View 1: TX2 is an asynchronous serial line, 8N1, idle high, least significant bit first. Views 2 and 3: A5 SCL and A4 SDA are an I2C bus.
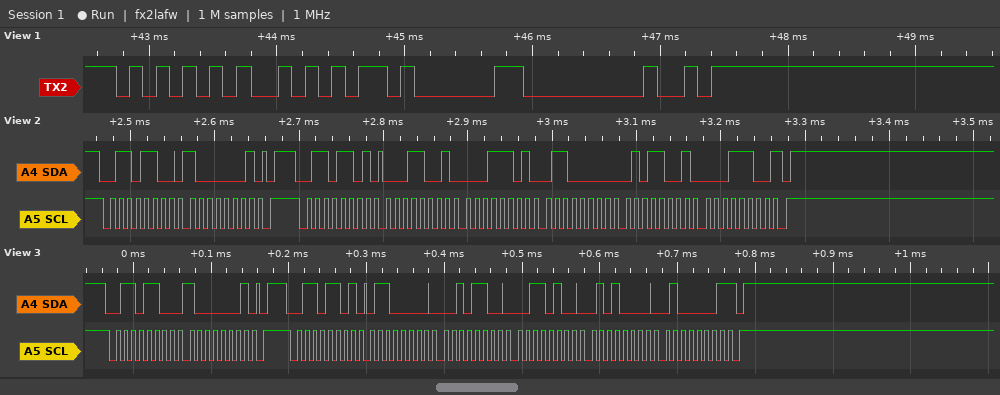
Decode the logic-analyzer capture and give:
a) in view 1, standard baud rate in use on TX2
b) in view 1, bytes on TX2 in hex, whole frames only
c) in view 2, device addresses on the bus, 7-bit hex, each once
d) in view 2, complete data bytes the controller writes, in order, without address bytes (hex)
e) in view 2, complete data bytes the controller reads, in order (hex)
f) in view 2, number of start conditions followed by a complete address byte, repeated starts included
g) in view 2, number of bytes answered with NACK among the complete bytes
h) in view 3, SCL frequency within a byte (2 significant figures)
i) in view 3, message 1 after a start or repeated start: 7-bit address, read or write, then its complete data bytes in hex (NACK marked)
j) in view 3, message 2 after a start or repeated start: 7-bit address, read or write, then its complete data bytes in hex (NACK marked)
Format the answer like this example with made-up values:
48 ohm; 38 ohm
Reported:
9600 baud; 55 AA 81 00 FA; 0x36; 81; 19 1D 60 59 1C; 2; 1; 100 kHz; 0x36 write: 81; 0x36 read: 60 2C 34 50 41 NACK
